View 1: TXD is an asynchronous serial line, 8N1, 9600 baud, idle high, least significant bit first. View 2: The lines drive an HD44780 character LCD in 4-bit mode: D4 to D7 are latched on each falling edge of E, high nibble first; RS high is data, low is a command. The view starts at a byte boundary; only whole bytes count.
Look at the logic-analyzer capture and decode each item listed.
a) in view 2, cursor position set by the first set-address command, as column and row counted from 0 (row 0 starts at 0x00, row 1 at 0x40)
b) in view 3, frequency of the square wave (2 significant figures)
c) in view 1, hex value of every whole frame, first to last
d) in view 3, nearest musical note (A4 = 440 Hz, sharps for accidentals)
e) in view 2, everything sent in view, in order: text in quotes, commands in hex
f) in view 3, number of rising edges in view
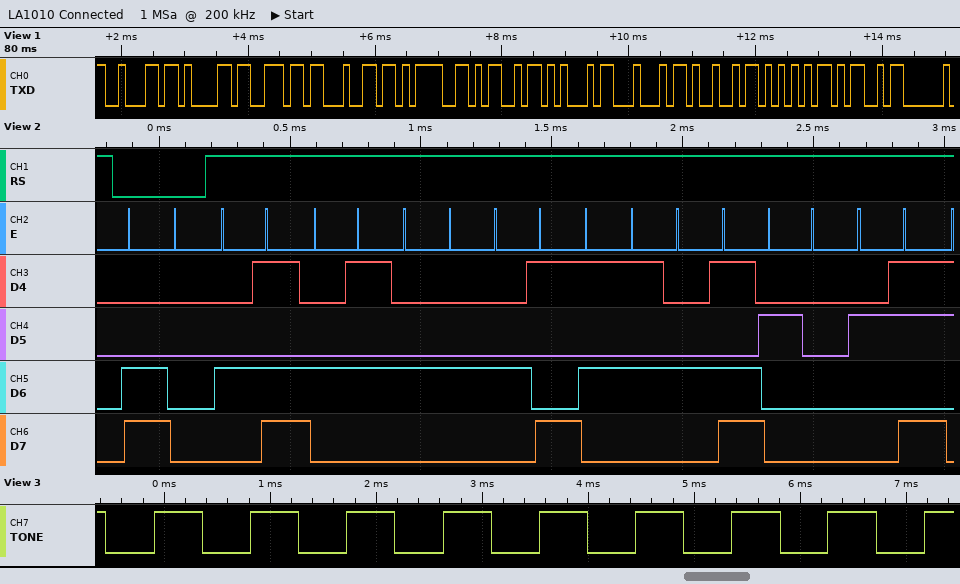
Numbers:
column 0, row 1
1.1 kHz
62 61 6E 64 3D 4D 45 44 49 55 4D
C#6
0xC0 "MEDIUM +"
9
